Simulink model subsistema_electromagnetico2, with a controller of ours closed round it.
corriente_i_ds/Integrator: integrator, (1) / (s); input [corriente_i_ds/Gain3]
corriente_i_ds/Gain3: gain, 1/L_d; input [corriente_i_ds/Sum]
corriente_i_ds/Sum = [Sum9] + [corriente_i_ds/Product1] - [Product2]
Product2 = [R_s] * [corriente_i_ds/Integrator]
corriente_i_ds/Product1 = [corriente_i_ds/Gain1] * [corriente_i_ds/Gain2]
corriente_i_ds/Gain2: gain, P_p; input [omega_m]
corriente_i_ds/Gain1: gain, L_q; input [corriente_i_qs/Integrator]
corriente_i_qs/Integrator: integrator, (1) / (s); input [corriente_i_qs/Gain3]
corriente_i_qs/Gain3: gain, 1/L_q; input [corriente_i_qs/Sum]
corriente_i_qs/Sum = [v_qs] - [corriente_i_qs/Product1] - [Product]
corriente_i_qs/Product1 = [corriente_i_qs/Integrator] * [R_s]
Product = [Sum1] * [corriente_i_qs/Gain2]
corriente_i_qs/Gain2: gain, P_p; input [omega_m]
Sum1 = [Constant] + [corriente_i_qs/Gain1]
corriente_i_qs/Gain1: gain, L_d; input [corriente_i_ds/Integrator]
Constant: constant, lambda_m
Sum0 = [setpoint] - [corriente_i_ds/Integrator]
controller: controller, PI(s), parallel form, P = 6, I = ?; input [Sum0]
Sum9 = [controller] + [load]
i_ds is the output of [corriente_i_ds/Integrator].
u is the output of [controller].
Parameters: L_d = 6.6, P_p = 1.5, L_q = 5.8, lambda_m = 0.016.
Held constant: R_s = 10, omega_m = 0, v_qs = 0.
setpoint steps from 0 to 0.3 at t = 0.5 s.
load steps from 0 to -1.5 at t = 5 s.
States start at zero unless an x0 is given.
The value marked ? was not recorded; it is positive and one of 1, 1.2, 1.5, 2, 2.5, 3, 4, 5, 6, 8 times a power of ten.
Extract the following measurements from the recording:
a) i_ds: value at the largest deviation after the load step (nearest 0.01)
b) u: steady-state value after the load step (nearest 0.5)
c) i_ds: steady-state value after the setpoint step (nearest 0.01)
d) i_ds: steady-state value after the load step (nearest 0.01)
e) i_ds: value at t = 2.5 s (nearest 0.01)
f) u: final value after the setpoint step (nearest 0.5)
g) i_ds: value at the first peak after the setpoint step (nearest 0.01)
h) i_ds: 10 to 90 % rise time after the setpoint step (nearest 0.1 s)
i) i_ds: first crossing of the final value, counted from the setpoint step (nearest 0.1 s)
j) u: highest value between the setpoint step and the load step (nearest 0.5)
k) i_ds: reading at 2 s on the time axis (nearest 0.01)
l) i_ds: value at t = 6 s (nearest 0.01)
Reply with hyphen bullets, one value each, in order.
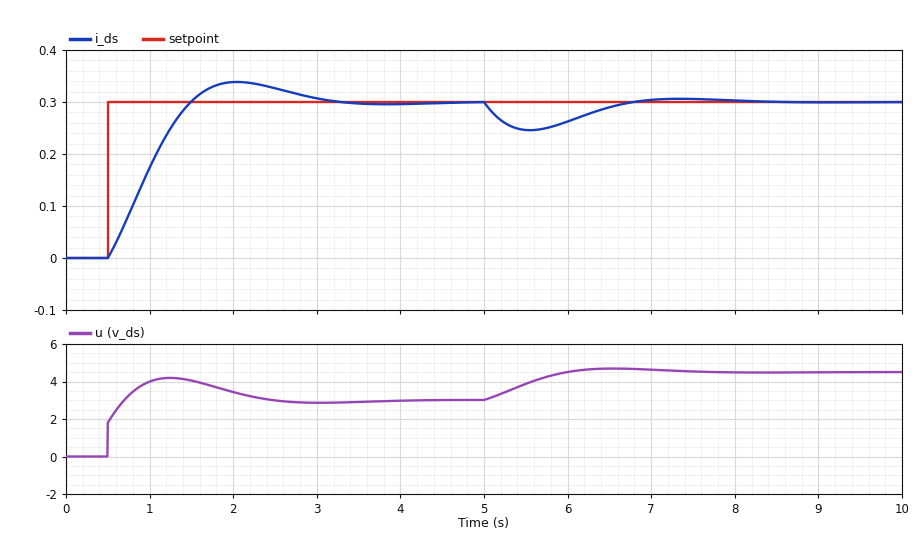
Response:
- 0.25
- 4.5
- 0.30
- 0.30
- 0.33
- 3.0
- 0.34
- 0.7 s
- 1.0 s
- 4.0
- 0.34
- 0.26
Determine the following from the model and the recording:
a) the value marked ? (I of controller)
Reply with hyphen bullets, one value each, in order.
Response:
- 30
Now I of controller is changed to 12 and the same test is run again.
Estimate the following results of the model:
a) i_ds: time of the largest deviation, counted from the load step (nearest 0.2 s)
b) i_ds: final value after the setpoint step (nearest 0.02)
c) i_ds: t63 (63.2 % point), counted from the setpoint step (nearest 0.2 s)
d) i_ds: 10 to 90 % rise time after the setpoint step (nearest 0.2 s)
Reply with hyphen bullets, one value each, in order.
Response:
- 0.8 s
- 0.30
- 1.0 s
- 1.8 s
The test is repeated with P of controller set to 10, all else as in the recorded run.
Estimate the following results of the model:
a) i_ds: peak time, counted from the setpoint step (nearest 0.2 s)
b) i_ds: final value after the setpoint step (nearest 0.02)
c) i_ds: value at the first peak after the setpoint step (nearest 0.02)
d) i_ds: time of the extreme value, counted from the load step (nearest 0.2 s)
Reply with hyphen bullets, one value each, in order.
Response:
- 1.6 s
- 0.30
- 0.32
- 0.6 s
